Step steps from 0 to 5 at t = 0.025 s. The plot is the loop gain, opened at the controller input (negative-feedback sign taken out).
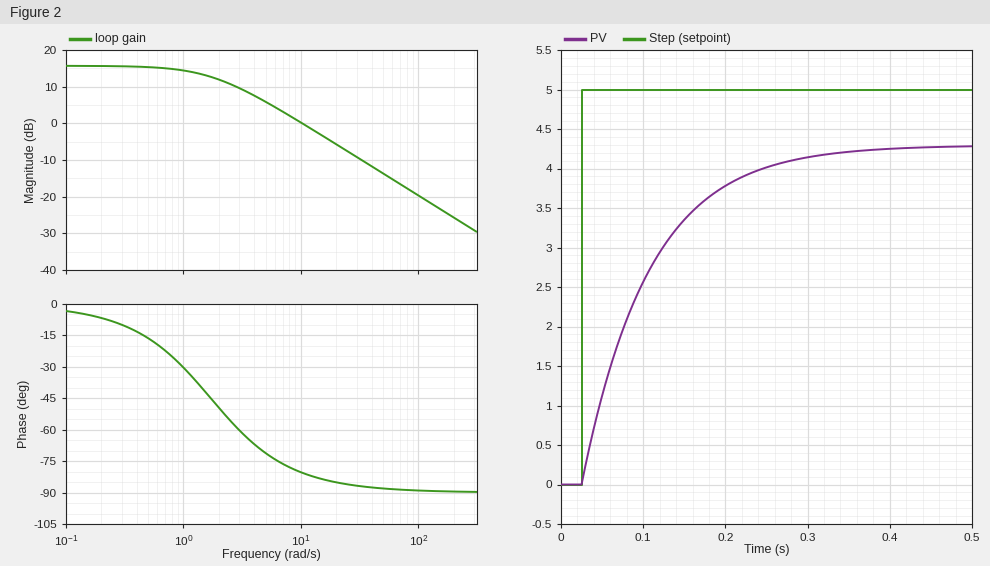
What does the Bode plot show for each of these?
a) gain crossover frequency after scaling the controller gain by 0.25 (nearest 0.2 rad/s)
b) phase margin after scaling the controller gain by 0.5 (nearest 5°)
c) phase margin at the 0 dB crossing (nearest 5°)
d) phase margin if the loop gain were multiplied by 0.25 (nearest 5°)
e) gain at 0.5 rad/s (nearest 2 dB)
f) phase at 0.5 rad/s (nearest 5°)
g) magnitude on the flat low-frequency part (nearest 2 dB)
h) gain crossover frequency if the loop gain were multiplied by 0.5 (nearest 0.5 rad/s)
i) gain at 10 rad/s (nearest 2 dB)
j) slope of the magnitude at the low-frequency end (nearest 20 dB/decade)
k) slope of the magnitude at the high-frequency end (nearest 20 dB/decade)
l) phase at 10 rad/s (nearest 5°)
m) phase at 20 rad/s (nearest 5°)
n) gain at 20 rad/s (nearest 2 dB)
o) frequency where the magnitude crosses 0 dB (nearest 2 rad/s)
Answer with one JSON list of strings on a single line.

["2.0 rad/s", "110°", "100°", "130°", "16 dB", "-15°", "16 dB", "5.0 rad/s", "0 dB", "0 dB/decade", "-20 dB/decade", "-80°", "-85°", "-6 dB", "10 rad/s"]
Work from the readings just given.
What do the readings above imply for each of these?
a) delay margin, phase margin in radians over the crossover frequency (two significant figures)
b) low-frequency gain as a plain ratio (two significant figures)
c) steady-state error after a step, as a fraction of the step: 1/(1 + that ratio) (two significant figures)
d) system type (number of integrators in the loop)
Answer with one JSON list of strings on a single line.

["0.17 s", "6.3", "0.14", "0"]
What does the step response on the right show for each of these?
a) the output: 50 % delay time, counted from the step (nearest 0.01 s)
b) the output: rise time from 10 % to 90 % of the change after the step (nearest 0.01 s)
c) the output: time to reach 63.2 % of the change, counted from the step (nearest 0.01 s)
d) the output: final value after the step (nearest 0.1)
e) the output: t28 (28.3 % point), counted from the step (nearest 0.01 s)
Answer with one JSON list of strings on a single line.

["0.06 s", "0.18 s", "0.08 s", "4.3", "0.03 s"]
